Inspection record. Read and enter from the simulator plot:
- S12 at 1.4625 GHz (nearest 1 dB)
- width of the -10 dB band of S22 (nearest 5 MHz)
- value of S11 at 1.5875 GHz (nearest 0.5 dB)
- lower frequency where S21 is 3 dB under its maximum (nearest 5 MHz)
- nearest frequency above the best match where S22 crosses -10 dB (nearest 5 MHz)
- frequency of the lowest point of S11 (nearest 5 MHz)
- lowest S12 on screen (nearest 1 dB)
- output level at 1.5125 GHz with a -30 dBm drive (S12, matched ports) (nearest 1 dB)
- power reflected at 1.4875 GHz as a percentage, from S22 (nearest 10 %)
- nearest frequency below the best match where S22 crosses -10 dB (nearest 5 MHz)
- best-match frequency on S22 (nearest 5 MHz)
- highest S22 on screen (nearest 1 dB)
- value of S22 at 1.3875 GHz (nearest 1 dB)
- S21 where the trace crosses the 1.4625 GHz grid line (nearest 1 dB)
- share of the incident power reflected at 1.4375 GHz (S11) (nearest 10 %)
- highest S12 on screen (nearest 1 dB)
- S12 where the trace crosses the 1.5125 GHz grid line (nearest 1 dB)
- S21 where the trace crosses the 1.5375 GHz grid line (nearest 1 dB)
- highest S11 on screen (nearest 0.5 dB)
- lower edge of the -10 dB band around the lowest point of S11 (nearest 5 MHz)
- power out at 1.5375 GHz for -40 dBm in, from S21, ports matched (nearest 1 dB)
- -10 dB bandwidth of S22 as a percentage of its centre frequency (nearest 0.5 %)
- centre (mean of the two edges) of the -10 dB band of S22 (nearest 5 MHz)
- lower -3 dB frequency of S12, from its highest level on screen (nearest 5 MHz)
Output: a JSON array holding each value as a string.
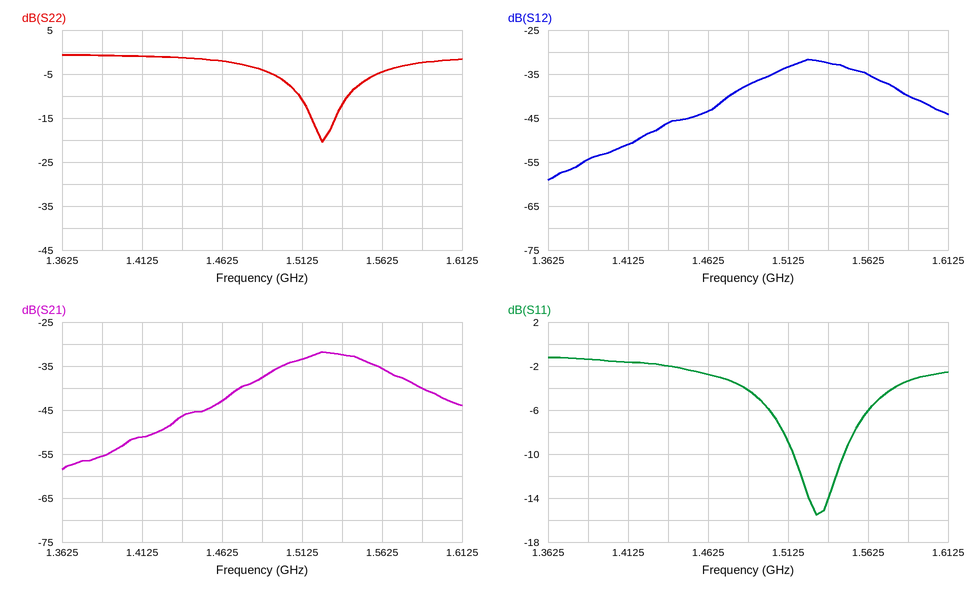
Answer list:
["-43 dB", "30 MHz", "-3.5 dB", "1.500 GHz", "1.540 GHz", "1.530 GHz", "-59 dB", "-63 dBm", "40 %", "1.510 GHz", "1.525 GHz", "-1 dB", "-1 dB", "-43 dB", "60 %", "-32 dB", "-33 dB", "-32 dB", "-1.0 dB", "1.515 GHz", "-72 dBm", "2.0 %", "1.525 GHz", "1.505 GHz"]
